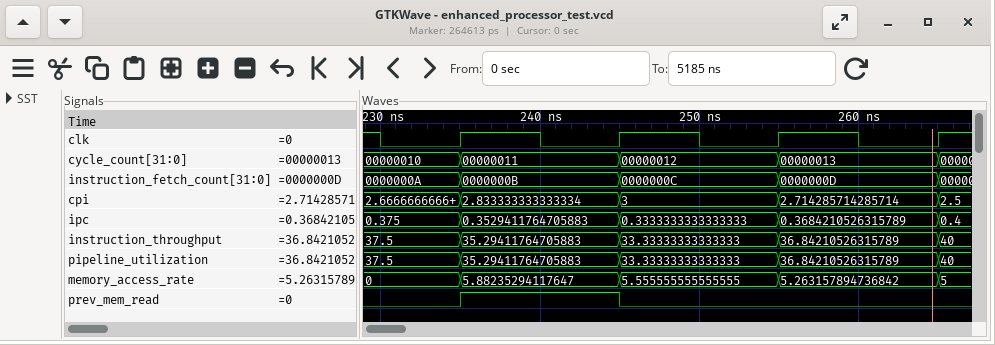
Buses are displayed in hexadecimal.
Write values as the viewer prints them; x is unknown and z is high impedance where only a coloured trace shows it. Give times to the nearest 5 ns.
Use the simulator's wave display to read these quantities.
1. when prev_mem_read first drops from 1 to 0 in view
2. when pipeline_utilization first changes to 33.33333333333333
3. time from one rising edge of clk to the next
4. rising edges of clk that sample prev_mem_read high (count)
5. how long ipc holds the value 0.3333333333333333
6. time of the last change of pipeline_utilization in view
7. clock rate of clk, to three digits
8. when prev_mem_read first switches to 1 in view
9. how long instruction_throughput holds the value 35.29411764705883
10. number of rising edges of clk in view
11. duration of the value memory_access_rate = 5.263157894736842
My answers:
245 ns
245 ns
10 ns
1
10 ns
265 ns
100 MHz
235 ns
10 ns
4
10 ns
